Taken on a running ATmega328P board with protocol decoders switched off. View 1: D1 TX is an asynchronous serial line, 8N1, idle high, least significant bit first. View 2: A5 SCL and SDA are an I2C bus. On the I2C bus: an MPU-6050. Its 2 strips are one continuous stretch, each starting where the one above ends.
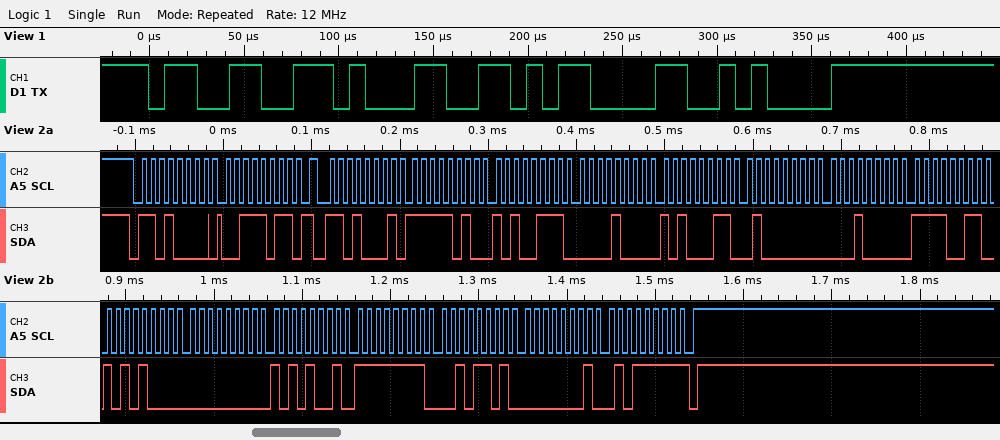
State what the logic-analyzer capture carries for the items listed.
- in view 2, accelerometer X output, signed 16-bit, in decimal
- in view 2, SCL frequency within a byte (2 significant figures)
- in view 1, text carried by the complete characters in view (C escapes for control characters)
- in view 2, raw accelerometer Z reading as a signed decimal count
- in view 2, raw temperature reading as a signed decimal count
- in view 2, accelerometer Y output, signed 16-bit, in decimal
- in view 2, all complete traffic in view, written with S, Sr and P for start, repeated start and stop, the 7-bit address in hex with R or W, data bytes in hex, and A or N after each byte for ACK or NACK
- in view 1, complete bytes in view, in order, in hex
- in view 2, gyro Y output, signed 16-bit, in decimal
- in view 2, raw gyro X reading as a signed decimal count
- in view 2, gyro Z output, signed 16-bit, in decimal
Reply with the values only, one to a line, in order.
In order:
-1369
100 kHz
"31\r\n"
16400
-3160
2211
S 68W A 3B A Sr 68R A FA A A7 A 08 A A3 A 40 A 10 A F3 A A8 A 00 A A9 A FF A 2D A 01 A 5F N P
33 31 0D 0A
-211
169
351
